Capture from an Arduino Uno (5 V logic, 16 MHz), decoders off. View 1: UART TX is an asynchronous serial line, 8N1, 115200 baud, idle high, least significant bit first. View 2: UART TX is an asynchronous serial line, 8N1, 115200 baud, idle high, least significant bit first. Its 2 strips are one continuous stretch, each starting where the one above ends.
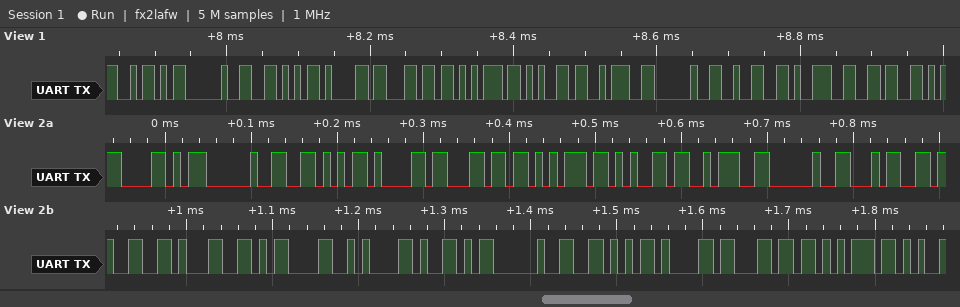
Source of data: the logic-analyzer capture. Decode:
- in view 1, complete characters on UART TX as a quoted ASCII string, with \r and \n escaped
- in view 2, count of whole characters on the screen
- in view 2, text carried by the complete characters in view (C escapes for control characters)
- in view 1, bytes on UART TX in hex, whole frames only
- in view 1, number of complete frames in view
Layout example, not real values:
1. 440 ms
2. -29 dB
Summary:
1. "Z Value: 296"
2. 20
3. "X Value: 431\r\nY Valu"
4. 0x5A 0x20 0x56 0x61 0x6C 0x75 0x65 0x3A 0x20 0x32 0x39 0x36
5. 12
